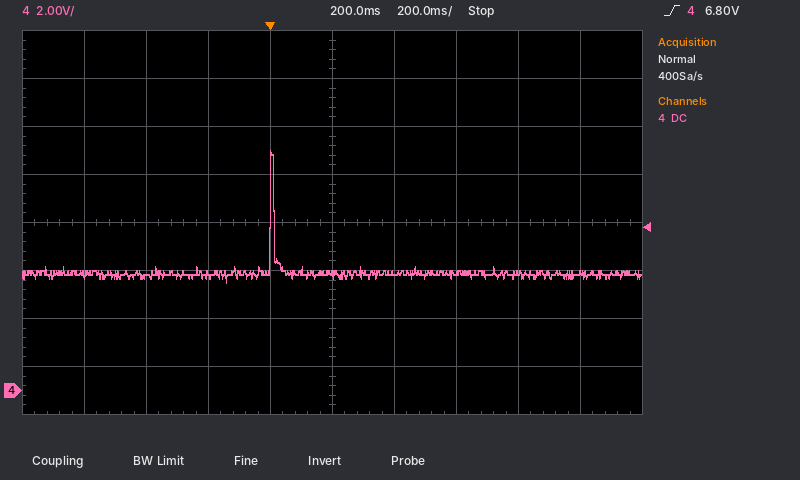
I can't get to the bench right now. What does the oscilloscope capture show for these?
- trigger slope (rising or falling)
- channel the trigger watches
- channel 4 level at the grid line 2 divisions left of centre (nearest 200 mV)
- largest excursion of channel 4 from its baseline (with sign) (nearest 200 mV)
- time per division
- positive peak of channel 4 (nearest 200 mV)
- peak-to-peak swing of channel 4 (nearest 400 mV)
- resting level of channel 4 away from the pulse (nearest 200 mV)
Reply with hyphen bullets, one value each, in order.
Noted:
- rising
- channel 4
- 4.8 V
- +5.2 V
- 200 ms
- 10.0 V
- 5.6 V
- 4.8 V
